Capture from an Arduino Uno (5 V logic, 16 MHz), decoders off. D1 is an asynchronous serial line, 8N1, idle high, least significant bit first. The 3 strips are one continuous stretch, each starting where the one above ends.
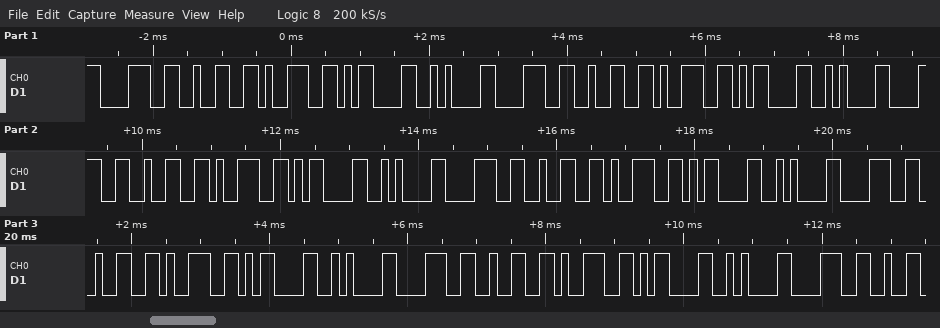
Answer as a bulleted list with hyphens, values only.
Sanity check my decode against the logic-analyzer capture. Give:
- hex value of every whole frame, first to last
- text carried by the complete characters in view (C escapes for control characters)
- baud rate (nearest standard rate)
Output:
- 38 32 39 0D 0A 38 32 39 0D 0A 38 32 39 0D 0A 38 32 39 0D 0A 38 32 39 0D 0A 38 32 39 0D 0A 38
- "829\r\n829\r\n829\r\n829\r\n829\r\n829\r\n8"
- 9600 baud
